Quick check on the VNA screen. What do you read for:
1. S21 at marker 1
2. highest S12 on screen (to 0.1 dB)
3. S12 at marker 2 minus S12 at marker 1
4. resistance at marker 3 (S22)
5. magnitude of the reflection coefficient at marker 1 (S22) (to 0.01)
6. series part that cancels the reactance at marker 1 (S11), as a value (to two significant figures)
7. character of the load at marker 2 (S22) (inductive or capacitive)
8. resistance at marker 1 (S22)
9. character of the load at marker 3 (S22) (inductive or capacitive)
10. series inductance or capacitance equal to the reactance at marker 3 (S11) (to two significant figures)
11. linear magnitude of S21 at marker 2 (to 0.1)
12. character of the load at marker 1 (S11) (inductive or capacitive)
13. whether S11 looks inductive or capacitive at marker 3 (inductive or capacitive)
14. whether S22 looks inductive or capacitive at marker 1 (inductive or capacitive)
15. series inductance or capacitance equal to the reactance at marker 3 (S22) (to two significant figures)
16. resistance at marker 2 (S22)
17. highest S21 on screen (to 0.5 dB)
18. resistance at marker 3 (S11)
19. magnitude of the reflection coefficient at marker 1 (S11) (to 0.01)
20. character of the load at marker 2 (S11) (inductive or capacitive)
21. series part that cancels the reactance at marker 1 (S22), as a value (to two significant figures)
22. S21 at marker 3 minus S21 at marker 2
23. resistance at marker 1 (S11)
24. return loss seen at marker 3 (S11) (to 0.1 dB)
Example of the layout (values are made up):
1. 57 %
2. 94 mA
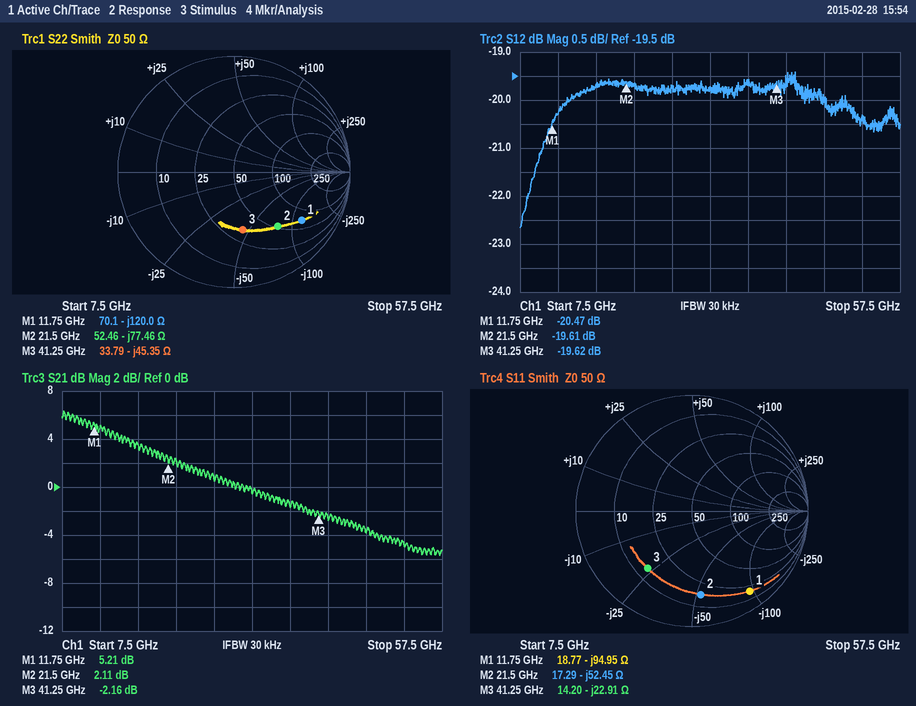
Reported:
1. 5.21 dB
2. -19.4 dB
3. 0.86 dB
4. 33.79 Ω
5. 0.72
6. 1.3 nH
7. capacitive
8. 70.1 Ω
9. capacitive
10. 170 fF
11. 1.3
12. capacitive
13. capacitive
14. capacitive
15. 85 fF
16. 52.46 Ω
17. 6.5 dB
18. 14.20 Ω
19. 0.85
20. capacitive
21. 1.6 nH
22. -4.27 dB
23. 18.77 Ω
24. 4.1 dB
